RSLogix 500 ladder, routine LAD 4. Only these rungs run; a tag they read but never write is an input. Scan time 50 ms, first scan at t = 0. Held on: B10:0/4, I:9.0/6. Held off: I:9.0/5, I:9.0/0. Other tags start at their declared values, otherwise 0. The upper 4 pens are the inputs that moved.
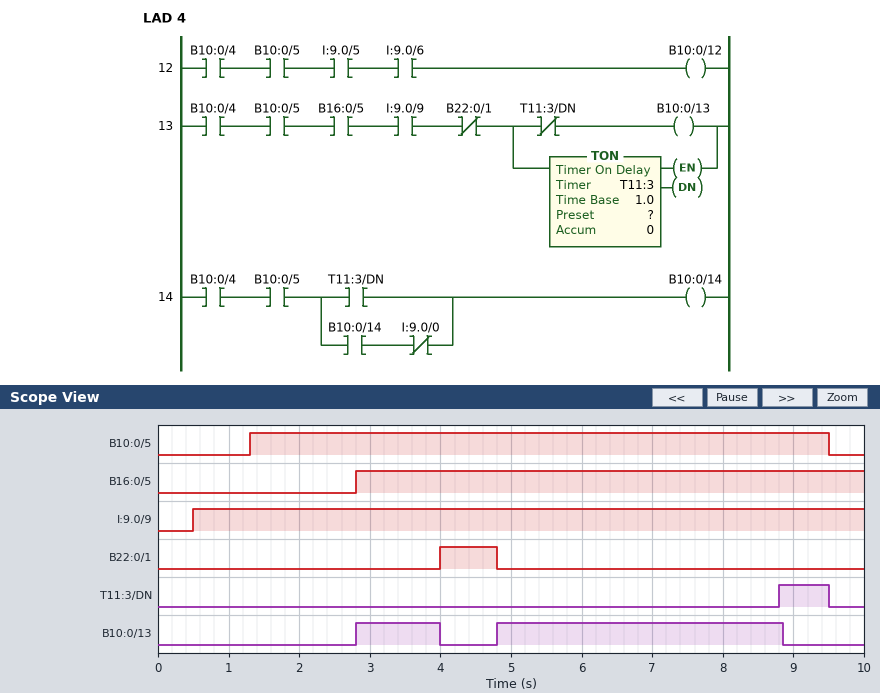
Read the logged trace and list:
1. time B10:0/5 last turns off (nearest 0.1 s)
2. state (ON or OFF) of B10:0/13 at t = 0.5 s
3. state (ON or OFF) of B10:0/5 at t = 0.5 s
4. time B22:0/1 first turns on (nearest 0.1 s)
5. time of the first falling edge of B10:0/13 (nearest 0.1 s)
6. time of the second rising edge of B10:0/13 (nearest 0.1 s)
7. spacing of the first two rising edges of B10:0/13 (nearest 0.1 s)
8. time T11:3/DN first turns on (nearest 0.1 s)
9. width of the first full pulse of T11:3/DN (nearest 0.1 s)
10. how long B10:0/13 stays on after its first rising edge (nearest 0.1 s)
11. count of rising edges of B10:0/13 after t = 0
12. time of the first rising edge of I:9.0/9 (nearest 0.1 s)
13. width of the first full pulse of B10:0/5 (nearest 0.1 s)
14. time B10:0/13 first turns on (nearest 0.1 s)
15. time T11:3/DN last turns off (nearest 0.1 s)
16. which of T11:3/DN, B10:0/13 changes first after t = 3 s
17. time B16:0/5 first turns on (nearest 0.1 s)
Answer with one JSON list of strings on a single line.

["9.5 s", "OFF", "OFF", "4.0 s", "4.0 s", "4.8 s", "2.0 s", "8.8 s", "0.7 s", "1.2 s", "2", "0.5 s", "8.2 s", "2.8 s", "9.5 s", "B10:0/13", "2.8 s"]
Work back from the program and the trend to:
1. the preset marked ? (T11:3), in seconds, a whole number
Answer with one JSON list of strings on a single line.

["4 s"]
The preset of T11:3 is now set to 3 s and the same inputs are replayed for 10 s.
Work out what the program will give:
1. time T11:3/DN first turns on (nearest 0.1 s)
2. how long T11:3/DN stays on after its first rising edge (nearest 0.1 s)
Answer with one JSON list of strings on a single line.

["7.8 s", "1.7 s"]
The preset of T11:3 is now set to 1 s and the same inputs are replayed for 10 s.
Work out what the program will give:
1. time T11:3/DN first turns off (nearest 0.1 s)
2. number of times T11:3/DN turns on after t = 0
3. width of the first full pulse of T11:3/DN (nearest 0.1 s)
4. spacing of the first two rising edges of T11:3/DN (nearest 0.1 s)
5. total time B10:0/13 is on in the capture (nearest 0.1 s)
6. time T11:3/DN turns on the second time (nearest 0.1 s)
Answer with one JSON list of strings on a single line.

["4.0 s", "2", "0.2 s", "2.0 s", "2.1 s", "5.8 s"]
